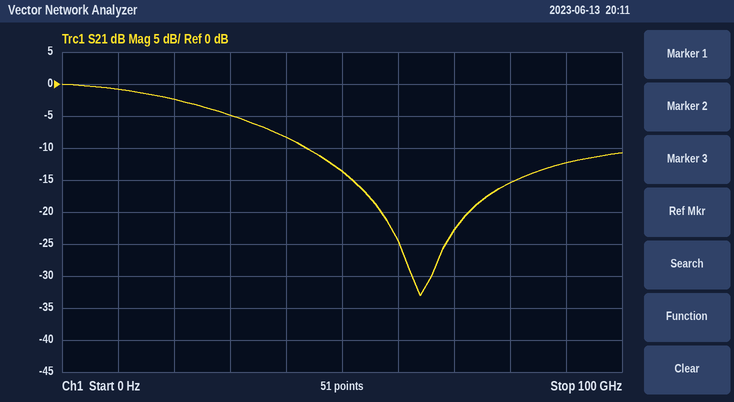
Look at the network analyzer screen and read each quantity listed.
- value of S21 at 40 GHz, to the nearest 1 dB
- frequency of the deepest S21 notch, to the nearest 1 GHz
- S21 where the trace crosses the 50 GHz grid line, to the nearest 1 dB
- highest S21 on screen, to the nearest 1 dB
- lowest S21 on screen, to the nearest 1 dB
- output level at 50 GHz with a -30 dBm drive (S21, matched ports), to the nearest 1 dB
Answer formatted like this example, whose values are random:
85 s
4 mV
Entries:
-8 dB
64 GHz
-14 dB
0 dB
-33 dB
-44 dBm
